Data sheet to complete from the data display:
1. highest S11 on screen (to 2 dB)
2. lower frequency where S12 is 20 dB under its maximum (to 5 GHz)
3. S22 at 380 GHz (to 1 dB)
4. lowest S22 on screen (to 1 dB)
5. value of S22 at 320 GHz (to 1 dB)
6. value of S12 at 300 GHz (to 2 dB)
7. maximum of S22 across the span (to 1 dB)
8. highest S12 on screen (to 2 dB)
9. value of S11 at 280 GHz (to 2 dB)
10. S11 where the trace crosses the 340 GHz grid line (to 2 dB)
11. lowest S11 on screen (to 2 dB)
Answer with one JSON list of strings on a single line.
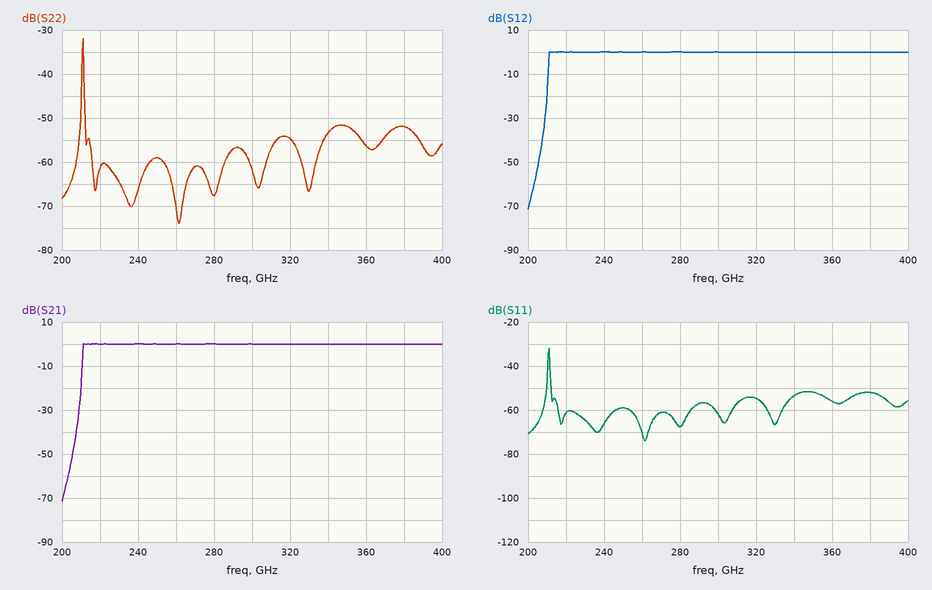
["-32 dB", "210 GHz", "-52 dB", "-74 dB", "-55 dB", "0 dB", "-32 dB", "0 dB", "-68 dB", "-54 dB", "-74 dB"]
